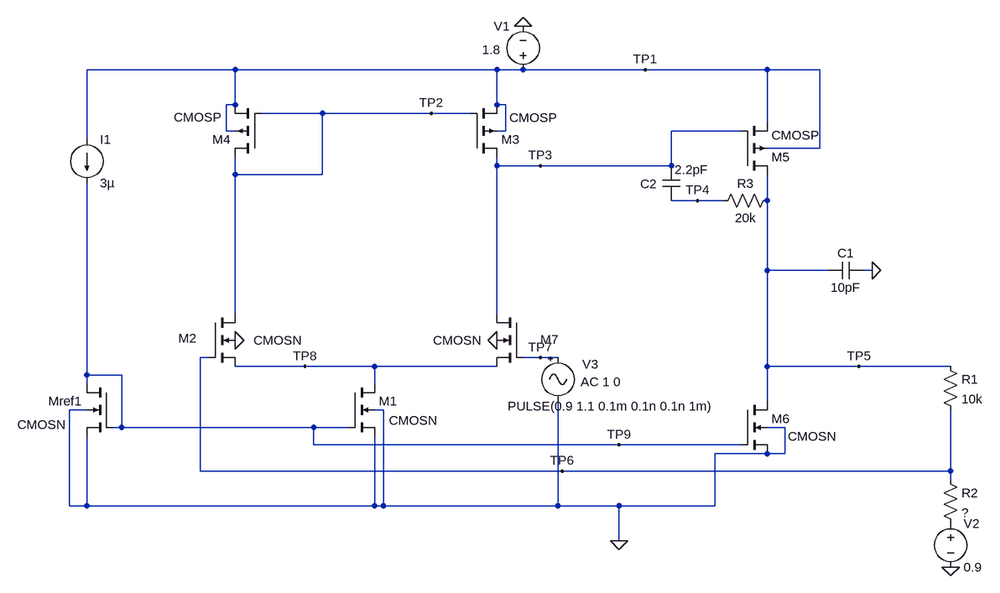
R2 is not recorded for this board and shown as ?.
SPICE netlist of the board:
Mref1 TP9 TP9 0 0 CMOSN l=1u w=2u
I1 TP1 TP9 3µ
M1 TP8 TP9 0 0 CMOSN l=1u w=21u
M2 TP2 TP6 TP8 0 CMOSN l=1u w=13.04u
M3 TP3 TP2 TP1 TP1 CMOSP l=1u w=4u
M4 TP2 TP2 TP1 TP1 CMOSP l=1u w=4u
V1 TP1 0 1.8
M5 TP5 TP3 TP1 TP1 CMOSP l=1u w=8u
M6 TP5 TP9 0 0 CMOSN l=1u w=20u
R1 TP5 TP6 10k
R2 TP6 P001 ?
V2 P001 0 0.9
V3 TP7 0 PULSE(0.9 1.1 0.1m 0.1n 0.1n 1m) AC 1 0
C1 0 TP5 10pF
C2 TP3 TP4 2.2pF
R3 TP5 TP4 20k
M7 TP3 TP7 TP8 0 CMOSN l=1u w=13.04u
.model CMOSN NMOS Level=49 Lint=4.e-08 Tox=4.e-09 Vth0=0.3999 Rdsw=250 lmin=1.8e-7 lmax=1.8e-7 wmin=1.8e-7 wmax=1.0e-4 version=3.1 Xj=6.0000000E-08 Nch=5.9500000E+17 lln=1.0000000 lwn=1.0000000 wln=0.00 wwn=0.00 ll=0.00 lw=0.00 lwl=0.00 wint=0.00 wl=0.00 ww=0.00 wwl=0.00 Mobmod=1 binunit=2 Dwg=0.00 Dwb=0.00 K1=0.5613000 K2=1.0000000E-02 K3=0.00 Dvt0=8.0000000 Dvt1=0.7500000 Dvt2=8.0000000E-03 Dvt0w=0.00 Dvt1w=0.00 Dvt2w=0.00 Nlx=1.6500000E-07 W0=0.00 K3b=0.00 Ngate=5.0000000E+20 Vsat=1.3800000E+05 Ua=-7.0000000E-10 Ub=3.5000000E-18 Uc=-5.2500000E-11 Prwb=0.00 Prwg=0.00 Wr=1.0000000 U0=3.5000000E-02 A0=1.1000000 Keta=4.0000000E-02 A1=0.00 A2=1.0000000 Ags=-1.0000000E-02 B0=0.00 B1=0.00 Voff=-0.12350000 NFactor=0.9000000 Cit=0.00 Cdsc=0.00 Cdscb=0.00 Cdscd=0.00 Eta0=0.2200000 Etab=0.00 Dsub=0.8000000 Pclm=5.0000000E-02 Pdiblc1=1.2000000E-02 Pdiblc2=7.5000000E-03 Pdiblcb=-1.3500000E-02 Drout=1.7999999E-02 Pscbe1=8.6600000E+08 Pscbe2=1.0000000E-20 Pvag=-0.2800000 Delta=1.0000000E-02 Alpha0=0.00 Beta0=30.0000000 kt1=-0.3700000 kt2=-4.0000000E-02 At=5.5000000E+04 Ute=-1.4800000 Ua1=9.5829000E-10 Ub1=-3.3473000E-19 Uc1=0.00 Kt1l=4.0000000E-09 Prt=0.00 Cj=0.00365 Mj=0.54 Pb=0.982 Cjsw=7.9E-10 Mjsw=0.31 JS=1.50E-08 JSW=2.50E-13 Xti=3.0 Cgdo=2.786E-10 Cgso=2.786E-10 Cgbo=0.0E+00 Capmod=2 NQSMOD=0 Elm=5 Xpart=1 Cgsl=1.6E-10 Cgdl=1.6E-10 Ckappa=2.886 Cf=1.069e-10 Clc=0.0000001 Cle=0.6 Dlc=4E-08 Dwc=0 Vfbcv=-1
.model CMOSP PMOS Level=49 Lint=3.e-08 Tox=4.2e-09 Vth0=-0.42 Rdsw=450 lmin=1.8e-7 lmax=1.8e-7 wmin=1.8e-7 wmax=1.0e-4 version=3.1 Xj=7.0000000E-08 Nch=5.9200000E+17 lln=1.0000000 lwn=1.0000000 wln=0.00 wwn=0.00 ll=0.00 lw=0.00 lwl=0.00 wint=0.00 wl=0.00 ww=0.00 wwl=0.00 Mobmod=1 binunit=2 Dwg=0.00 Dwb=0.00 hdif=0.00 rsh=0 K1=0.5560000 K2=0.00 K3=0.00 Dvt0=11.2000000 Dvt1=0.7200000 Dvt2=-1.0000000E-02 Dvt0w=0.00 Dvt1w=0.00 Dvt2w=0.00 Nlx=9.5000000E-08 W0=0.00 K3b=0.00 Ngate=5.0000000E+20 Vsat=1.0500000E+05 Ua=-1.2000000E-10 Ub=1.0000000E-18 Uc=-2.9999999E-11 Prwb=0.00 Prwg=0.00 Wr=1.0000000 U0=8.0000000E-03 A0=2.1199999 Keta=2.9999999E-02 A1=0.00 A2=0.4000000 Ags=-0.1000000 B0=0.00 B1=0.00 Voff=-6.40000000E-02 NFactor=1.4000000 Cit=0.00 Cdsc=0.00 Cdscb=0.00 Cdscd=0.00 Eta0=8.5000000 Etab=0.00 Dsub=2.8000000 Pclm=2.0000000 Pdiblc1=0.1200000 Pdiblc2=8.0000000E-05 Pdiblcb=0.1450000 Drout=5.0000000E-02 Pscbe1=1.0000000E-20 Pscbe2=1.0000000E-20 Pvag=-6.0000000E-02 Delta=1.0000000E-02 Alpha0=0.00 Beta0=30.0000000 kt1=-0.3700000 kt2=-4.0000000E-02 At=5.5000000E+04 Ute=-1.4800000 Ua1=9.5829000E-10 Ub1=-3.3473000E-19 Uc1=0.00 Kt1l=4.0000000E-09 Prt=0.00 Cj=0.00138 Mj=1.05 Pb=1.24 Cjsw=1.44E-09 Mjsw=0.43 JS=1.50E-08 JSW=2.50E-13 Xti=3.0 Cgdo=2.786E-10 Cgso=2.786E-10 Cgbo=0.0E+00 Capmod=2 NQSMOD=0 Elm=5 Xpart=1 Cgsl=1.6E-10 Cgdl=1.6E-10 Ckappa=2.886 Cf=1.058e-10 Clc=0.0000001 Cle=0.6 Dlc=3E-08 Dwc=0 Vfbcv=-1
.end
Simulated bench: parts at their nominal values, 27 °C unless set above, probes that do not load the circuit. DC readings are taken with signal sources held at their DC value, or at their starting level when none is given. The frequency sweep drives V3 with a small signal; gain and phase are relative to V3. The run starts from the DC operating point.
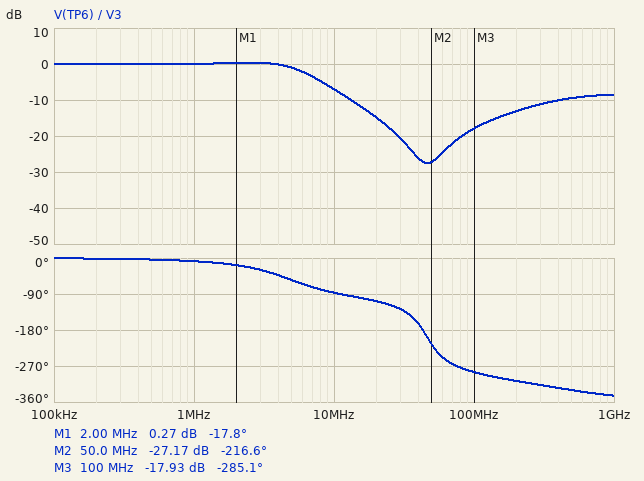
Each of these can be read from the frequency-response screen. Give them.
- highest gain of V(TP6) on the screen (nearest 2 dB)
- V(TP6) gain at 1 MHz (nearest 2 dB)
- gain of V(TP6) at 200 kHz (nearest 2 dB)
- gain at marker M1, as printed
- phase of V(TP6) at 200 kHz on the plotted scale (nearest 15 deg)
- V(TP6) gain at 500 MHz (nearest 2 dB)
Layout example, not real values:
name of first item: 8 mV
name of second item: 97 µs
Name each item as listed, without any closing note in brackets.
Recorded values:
highest gain of V(TP6) on the screen: 0 dB
V(TP6) gain at 1 MHz: 0 dB
gain of V(TP6) at 200 kHz: 0 dB
gain at marker M1, as printed: 0.27 dB
phase of V(TP6) at 200 kHz on the plotted scale: 0 deg
V(TP6) gain at 500 MHz: -10 dB
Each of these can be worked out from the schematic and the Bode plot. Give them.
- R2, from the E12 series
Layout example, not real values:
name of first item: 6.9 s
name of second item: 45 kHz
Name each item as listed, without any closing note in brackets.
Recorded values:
R2, from the E12 series: 18 kΩ
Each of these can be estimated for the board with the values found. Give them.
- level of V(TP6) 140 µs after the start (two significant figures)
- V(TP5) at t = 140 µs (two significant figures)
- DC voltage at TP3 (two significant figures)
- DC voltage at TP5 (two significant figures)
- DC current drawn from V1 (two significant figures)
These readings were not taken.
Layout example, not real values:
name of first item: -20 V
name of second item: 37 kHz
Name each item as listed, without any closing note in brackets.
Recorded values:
level of V(TP6) 140 µs after the start: 1.1 V
V(TP5) at t = 140 µs: 1.2 V
DC voltage at TP3: 950 mV
DC voltage at TP5: 900 mV
DC current drawn from V1: 65 µA
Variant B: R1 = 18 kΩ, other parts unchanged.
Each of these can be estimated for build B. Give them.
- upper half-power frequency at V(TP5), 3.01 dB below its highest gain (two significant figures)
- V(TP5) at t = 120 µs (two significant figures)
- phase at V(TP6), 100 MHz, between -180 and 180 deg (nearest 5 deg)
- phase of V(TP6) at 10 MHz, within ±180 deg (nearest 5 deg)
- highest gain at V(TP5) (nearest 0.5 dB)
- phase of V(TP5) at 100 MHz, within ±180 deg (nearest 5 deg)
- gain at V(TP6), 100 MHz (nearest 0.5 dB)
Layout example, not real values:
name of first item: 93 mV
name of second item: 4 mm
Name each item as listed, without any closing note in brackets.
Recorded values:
upper half-power frequency at V(TP5), 3.01 dB below its highest gain: 5.4 MHz
V(TP5) at t = 120 µs: 1.3 V
phase at V(TP6), 100 MHz, between -180 and 180 deg: 65 deg
phase of V(TP6) at 10 MHz, within ±180 deg: -95 deg
highest gain at V(TP5): 6.5 dB
phase of V(TP5) at 100 MHz, within ±180 deg: -165 deg
gain at V(TP6), 100 MHz: -15.0 dB
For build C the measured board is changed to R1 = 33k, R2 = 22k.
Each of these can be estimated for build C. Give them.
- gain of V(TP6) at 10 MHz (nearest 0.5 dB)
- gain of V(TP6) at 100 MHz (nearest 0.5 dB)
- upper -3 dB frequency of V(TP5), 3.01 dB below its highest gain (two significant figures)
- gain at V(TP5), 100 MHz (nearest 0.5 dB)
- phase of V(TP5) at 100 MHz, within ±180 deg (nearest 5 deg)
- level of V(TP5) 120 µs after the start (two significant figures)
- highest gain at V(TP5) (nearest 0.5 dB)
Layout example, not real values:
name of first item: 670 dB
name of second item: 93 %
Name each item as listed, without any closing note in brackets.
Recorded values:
gain of V(TP6) at 10 MHz: -11.5 dB
gain of V(TP6) at 100 MHz: -12.0 dB
upper -3 dB frequency of V(TP5), 3.01 dB below its highest gain: 4.7 MHz
gain at V(TP5), 100 MHz: -29.5 dB
phase of V(TP5) at 100 MHz, within ±180 deg: -165 deg
level of V(TP5) 120 µs after the start: 1.4 V
highest gain at V(TP5): 8.5 dB
